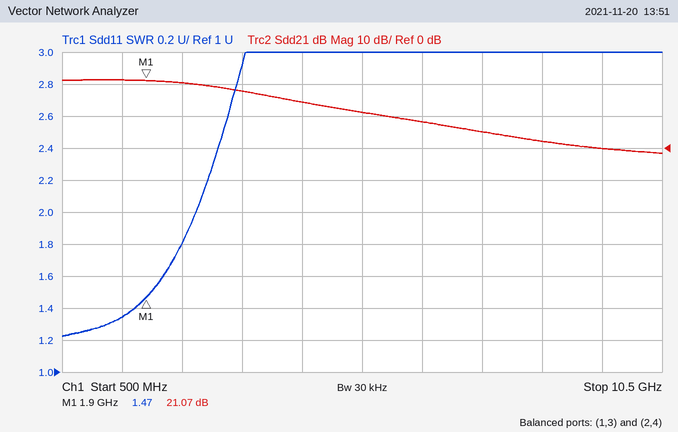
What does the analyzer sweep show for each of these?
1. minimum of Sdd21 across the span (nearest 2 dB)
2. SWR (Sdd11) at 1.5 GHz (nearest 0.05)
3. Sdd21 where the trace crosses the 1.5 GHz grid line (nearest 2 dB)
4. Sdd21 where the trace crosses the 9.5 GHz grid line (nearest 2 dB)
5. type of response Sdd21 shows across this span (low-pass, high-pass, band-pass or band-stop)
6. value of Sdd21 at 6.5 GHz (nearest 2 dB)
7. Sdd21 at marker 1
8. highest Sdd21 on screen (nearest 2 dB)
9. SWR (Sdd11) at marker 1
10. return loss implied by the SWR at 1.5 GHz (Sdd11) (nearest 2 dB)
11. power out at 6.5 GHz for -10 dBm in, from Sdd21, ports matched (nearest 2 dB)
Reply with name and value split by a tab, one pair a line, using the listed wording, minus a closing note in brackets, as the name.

minimum of Sdd21 across the span	-2 dB
SWR (Sdd11) at 1.5 GHz	1.35
Sdd21 where the trace crosses the 1.5 GHz grid line	22 dB
Sdd21 where the trace crosses the 9.5 GHz grid line	0 dB
type of response Sdd21 shows across this span	low-pass
value of Sdd21 at 6.5 GHz	8 dB
Sdd21 at marker 1	21.07 dB
highest Sdd21 on screen	22 dB
SWR (Sdd11) at marker 1	1.47
return loss implied by the SWR at 1.5 GHz (Sdd11)	16 dB
power out at 6.5 GHz for -10 dBm in, from Sdd21, ports matched	-2 dBm
